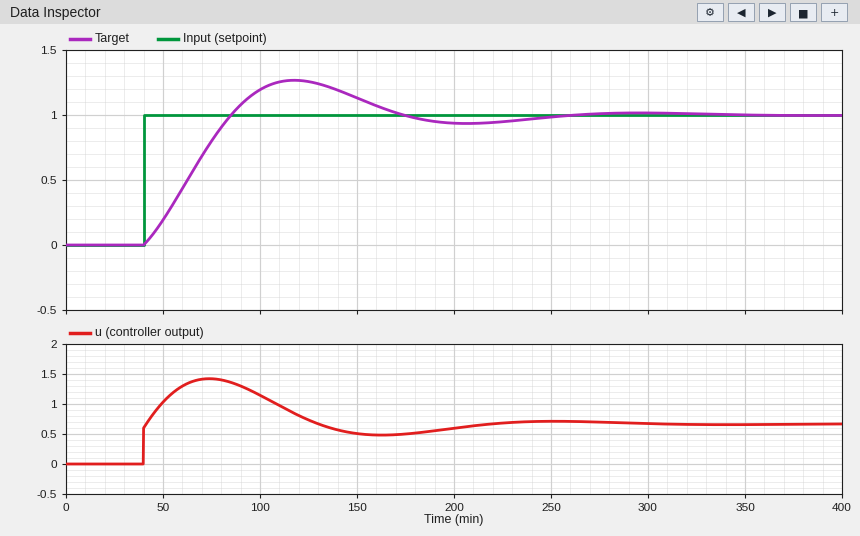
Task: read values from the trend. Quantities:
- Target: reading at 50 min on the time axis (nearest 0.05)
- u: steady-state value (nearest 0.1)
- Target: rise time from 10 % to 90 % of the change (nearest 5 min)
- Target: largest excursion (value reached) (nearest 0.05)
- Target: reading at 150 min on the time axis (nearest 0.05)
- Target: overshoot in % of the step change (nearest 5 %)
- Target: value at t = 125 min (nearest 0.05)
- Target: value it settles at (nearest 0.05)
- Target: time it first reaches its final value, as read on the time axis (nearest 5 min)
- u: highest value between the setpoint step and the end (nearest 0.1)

0.20
0.7
35 min
1.25
1.15
25 %
1.25
1.00
85 min
1.4
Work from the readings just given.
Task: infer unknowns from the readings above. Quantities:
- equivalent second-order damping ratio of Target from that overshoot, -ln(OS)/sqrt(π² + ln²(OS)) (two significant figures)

0.40
